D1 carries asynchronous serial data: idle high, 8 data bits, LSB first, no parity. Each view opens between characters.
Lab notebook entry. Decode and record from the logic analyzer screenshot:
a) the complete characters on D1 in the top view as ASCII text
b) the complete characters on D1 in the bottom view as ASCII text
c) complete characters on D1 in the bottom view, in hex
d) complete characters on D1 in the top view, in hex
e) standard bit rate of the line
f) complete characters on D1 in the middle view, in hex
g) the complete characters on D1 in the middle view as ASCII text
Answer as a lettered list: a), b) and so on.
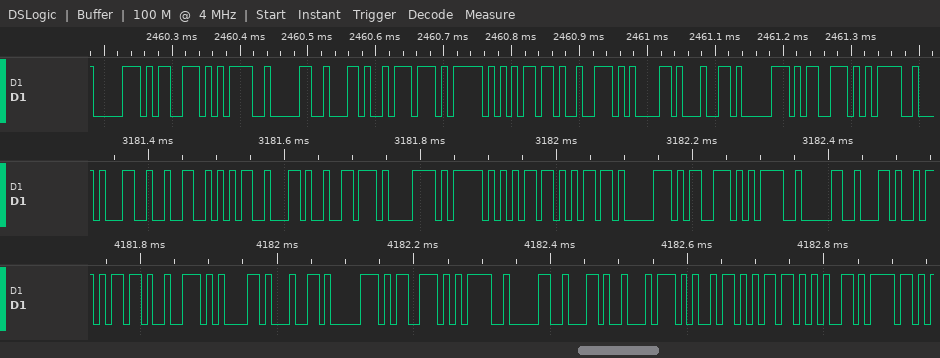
a) "ps=0,w_mradps="
b) "mradps=0,timeo"
c) 6D, 72, 61, 64, 70, 73, 3D, 30, 2C, 74, 69, 6D, 65, 6F
d) 70, 73, 3D, 30, 2C, 77, 5F, 6D, 72, 61, 64, 70, 73, 3D
e) 115200 baud
f) 31, 32, 35, 2C, 76, 78, 5F, 6D, 6D, 70, 73, 3D, 30, 2C
g) "125,vx_mmps=0,"
